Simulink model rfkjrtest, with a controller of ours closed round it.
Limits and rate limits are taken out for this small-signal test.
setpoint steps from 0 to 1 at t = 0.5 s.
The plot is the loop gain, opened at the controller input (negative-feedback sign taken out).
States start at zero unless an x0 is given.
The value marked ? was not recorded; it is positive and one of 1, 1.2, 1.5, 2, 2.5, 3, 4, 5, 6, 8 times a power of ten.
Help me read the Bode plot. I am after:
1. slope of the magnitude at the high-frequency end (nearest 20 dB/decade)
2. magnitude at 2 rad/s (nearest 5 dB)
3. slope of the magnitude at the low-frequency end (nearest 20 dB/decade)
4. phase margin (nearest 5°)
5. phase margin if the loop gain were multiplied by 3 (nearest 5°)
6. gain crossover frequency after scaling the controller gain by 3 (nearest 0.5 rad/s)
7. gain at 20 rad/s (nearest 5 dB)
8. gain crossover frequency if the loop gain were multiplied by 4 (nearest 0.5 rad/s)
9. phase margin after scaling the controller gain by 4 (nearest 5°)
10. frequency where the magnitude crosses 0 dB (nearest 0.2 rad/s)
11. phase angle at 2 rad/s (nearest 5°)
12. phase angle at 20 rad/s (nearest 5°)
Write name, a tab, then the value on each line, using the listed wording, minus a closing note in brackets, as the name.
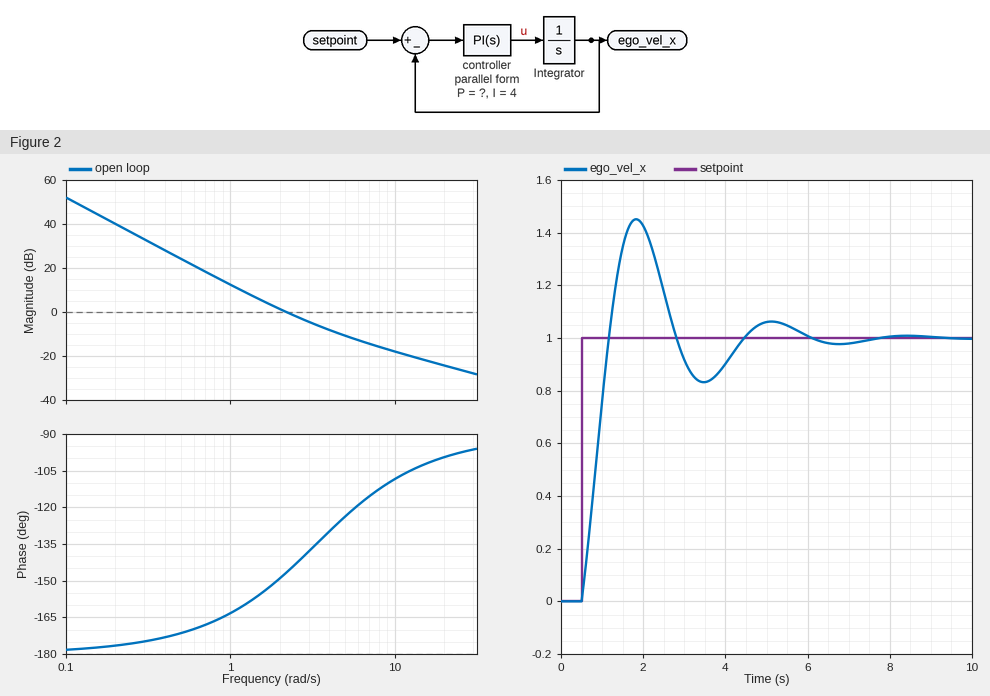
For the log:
slope of the magnitude at the high-frequency end	-20 dB/decade
magnitude at 2 rad/s	0 dB
slope of the magnitude at the low-frequency end	-40 dB/decade
phase margin	35°
phase margin if the loop gain were multiplied by 3	55°
gain crossover frequency after scaling the controller gain by 3	4.5 rad/s
gain at 20 rad/s	-25 dB
gain crossover frequency if the loop gain were multiplied by 4	5.5 rad/s
phase margin after scaling the controller gain by 4	60°
frequency where the magnitude crosses 0 dB	2.2 rad/s
phase angle at 2 rad/s	-150°
phase angle at 20 rad/s	-100°
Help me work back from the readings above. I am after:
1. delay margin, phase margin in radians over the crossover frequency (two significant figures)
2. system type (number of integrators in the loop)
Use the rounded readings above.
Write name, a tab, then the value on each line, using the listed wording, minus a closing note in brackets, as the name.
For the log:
delay margin, phase margin in radians over the crossover frequency	0.28 s
system type	2
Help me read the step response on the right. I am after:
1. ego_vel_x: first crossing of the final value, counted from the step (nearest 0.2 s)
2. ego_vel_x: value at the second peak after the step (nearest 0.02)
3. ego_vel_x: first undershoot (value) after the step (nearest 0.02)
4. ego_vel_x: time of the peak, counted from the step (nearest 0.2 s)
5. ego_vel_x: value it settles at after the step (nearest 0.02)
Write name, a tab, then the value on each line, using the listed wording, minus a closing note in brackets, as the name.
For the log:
ego_vel_x: first crossing of the final value, counted from the step	0.6 s
ego_vel_x: value at the second peak after the step	1.06
ego_vel_x: first undershoot (value) after the step	0.84
ego_vel_x: time of the peak, counted from the step	1.4 s
ego_vel_x: value it settles at after the step	1.00
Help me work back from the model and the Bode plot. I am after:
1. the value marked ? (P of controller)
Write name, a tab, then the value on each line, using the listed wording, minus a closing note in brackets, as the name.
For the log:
the value marked ?	1.2
